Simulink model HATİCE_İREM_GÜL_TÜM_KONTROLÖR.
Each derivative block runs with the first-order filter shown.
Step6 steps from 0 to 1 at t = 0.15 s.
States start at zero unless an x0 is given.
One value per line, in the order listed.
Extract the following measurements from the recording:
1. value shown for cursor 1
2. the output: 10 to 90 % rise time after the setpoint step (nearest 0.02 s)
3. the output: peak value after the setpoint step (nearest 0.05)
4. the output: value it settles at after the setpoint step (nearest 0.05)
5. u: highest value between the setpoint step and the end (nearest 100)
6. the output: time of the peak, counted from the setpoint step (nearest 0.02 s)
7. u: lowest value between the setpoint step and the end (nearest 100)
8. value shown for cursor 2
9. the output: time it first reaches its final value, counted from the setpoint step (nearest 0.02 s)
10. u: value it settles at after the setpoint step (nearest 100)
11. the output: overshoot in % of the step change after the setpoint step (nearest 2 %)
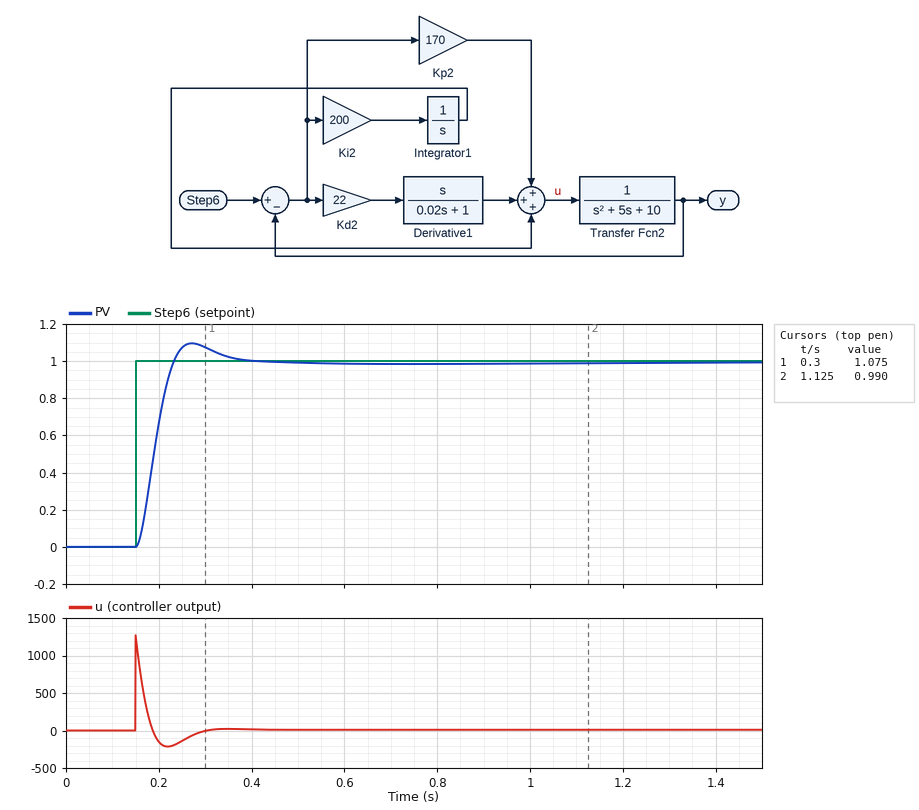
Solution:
1.075
0.06 s
1.10
1.00
1300
0.12 s
-200
0.990
0.08 s
0
10 %
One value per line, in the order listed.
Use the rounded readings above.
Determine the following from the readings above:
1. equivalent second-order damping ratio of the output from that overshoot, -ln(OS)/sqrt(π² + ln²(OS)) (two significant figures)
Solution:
0.59
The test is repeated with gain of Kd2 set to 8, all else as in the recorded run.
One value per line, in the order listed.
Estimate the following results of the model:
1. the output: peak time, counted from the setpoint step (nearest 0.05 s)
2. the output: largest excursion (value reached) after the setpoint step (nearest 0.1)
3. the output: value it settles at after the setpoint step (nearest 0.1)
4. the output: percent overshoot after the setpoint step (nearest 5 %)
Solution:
0.20 s
1.3
1.0
25 %
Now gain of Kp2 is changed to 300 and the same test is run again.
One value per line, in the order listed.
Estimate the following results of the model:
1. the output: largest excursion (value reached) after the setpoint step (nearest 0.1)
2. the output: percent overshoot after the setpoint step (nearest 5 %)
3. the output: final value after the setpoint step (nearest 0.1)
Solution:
1.2
20 %
1.0
